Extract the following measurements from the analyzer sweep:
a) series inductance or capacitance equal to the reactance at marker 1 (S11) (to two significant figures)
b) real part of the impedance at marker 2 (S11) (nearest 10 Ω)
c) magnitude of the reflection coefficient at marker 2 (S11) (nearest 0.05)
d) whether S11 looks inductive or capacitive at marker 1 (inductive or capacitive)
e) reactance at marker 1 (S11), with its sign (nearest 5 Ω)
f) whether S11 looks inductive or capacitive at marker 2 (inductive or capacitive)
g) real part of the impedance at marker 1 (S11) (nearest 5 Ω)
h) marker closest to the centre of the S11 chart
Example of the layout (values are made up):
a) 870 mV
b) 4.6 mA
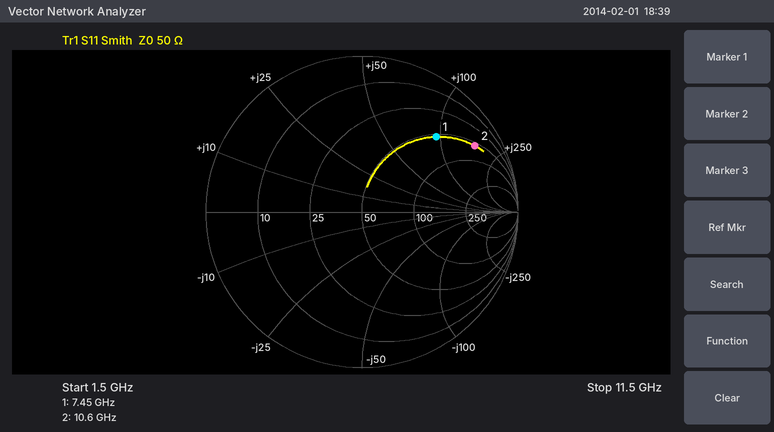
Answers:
a) 2.0 nH
b) 60 Ω
c) 0.85
d) inductive
e) +95 Ω
f) inductive
g) 55 Ω
h) marker 1
